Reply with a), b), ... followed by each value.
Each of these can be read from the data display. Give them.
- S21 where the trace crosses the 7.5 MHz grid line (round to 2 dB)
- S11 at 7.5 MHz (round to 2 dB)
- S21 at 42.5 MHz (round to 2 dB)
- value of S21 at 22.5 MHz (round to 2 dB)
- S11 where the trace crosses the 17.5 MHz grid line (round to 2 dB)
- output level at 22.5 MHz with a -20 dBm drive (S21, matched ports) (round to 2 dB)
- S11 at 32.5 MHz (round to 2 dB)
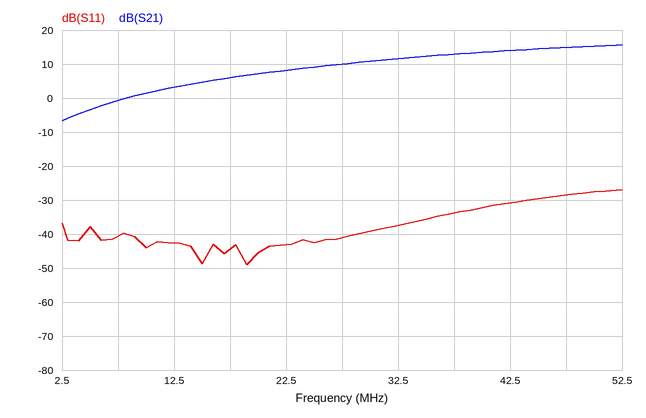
a) 0 dB
b) -40 dB
c) 14 dB
d) 8 dB
e) -44 dB
f) -12 dBm
g) -38 dB
